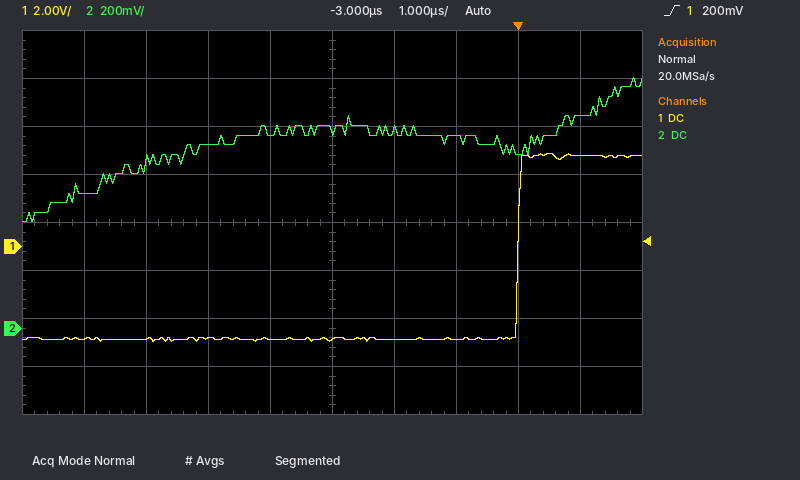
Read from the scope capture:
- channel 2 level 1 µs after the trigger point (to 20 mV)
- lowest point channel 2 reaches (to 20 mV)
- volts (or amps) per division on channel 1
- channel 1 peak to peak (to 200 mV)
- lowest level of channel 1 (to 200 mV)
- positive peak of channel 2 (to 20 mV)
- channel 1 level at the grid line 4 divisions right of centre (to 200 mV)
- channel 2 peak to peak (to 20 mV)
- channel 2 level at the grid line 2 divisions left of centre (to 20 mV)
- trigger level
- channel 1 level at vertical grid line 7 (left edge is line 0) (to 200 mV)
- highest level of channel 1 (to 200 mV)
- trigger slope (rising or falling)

880 mV
440 mV
2 V
7.8 V
-4.0 V
1.04 V
3.8 V
600 mV
760 mV
200 mV
-3.8 V
3.8 V
rising
